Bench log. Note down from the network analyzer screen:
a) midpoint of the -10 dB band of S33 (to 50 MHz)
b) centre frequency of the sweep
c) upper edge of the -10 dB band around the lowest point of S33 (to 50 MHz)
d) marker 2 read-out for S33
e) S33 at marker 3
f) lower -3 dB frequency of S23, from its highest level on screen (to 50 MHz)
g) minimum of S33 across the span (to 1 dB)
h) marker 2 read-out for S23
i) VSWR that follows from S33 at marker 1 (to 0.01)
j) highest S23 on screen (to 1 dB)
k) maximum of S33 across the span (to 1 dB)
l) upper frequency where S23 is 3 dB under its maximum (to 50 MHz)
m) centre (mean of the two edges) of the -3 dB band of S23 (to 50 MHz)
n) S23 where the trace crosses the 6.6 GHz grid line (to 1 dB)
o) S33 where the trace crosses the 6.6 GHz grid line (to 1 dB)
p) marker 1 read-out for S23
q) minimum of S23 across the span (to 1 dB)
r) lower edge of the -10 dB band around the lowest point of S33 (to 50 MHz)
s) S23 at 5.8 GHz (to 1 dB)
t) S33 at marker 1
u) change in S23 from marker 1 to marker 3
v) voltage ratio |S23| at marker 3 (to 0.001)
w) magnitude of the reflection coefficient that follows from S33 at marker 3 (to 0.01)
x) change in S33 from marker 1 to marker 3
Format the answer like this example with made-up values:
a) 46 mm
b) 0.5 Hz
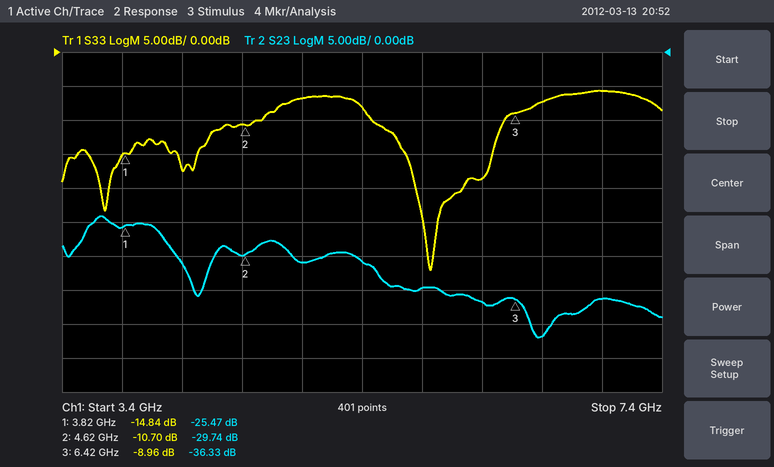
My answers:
a) 5.90 GHz
b) 5.4 GHz
c) 6.35 GHz
d) -10.70 dB
e) -8.96 dB
f) 3.55 GHz
g) -32 dB
h) -29.74 dB
i) 1.44
j) -24 dB
k) -6 dB
l) 4.05 GHz
m) 3.80 GHz
n) -42 dB
o) -7 dB
p) -25.47 dB
q) -42 dB
r) 5.45 GHz
s) -35 dB
t) -14.84 dB
u) -10.86 dB
v) 0.015
w) 0.36
x) 5.88 dB
